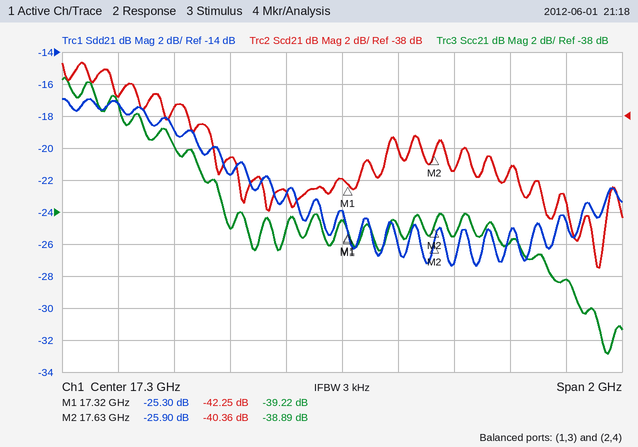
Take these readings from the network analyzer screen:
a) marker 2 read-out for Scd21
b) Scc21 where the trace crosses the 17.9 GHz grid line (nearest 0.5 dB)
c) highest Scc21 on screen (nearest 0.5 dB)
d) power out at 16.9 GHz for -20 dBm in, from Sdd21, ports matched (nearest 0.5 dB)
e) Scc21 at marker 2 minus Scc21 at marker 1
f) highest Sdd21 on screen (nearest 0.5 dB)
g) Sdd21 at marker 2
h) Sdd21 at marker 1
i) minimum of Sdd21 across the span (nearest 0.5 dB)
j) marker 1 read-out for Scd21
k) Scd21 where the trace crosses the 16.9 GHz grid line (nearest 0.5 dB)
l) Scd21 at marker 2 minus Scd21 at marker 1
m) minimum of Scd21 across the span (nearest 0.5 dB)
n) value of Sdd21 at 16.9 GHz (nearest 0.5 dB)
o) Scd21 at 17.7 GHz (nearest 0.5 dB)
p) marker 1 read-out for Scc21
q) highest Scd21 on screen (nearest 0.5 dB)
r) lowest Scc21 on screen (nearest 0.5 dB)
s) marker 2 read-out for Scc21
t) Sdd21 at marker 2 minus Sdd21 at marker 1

-40.36 dB
-40.0 dB
-29.5 dB
-41.5 dBm
0.33 dB
-17.0 dB
-25.90 dB
-25.30 dB
-27.5 dB
-42.25 dB
-40.5 dB
1.89 dB
-47.5 dB
-21.5 dB
-41.5 dB
-39.22 dB
-34.5 dB
-47.0 dB
-38.89 dB
-0.60 dB
